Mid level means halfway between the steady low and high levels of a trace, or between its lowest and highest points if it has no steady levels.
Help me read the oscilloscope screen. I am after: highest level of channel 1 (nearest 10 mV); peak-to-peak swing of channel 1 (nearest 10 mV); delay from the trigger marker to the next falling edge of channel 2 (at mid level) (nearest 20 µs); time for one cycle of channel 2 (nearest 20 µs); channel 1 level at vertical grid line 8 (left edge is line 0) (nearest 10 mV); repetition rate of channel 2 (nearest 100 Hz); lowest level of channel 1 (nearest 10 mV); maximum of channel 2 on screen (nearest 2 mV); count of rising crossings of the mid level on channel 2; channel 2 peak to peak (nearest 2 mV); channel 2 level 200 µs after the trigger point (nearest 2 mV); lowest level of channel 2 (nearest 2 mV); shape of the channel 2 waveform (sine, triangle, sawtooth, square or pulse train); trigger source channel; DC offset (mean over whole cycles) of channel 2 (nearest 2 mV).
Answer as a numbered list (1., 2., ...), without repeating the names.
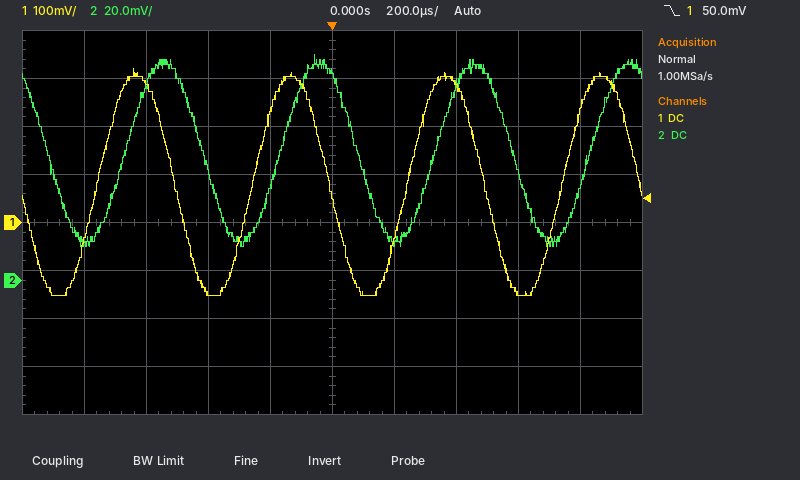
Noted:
1. 320 mV
2. 470 mV
3. 80 µs
4. 500 µs
5. -140 mV
6. 2.0 kHz
7. -150 mV
8. 94 mV
9. 4
10. 80 mV
11. 16 mV
12. 14 mV
13. sine
14. channel 1
15. 54 mV
